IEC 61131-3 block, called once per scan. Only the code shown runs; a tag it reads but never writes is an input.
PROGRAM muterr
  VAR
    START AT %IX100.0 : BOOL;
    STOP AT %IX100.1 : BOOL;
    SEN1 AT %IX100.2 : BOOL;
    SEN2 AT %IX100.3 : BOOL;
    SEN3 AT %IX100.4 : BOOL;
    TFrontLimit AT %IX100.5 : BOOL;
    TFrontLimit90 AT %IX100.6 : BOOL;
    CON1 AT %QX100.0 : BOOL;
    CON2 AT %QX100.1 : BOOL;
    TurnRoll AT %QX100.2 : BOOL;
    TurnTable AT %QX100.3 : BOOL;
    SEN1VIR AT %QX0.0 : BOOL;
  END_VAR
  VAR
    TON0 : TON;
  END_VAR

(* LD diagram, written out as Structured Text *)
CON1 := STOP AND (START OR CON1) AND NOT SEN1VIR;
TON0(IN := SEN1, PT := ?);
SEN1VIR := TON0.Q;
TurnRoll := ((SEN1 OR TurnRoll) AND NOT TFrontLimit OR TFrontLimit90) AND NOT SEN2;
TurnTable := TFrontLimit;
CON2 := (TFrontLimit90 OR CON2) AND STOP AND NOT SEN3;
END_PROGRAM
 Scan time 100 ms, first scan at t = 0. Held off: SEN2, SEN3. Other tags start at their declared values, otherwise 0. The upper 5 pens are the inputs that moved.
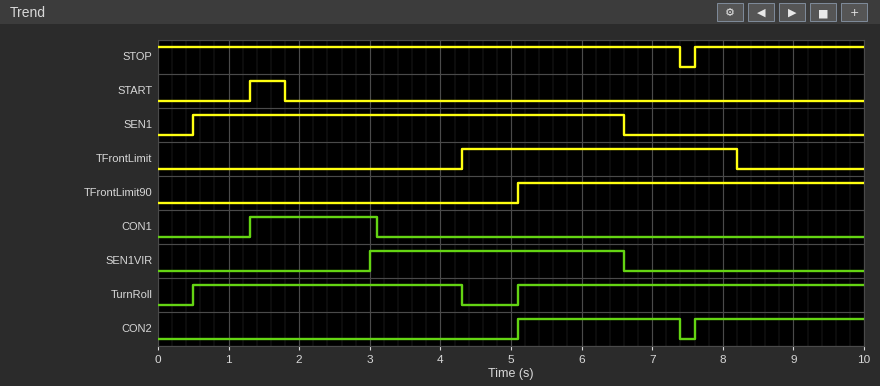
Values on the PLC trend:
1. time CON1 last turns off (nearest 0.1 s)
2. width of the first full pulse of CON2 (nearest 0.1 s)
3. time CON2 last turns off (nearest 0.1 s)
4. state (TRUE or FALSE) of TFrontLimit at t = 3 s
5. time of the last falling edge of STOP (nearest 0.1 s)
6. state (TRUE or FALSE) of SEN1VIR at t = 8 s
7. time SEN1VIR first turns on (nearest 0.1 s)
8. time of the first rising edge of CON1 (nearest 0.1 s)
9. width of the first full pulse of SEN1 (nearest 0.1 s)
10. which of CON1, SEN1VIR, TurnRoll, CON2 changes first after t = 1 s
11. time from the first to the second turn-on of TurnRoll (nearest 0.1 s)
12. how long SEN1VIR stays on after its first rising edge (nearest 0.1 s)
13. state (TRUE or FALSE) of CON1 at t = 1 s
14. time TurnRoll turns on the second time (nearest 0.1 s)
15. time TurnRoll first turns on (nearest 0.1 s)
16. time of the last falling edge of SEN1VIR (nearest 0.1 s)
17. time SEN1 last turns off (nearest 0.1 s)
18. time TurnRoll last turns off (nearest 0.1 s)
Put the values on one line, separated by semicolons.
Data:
3.1 s; 2.3 s; 7.4 s; FALSE; 7.4 s; FALSE; 3.0 s; 1.3 s; 6.1 s; CON1; 4.6 s; 3.6 s; FALSE; 5.1 s; 0.5 s; 6.6 s; 6.6 s; 4.3 s
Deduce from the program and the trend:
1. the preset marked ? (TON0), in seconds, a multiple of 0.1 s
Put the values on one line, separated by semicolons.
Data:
2.5 s
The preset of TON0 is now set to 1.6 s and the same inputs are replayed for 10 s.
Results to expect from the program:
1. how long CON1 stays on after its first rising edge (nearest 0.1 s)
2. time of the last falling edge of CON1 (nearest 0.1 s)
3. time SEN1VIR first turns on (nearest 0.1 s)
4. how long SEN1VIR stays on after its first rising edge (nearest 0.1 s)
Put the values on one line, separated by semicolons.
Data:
0.9 s; 2.2 s; 2.1 s; 4.5 s
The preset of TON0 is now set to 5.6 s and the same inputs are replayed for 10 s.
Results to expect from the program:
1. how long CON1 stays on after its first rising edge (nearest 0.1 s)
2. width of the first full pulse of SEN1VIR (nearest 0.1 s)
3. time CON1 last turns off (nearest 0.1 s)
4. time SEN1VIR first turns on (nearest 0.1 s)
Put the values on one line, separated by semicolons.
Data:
4.9 s; 0.5 s; 6.2 s; 6.1 s
